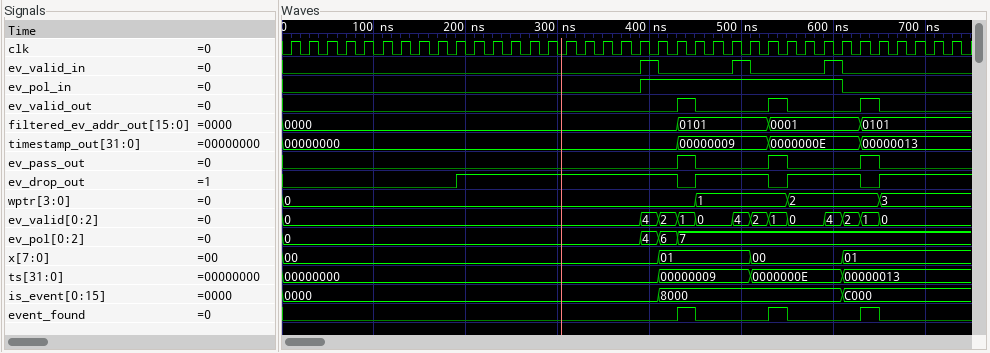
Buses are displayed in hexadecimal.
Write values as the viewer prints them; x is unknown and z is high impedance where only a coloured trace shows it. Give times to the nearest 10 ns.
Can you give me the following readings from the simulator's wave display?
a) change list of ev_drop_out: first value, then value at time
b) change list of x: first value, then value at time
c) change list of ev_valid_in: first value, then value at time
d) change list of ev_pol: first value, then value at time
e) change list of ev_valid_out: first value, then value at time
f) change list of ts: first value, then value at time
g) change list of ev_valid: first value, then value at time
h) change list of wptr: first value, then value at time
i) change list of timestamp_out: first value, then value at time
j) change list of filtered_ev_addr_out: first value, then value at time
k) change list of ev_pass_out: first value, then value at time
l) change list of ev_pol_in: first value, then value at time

0, 1 at 190 ns, 0 at 430 ns, 1 at 450 ns, 0 at 530 ns, 1 at 550 ns, 0 at 630 ns, 1 at 650 ns
00, 01 at 410 ns, 00 at 510 ns, 01 at 610 ns
0, 1 at 390 ns, 0 at 410 ns, 1 at 490 ns, 0 at 510 ns, 1 at 590 ns, 0 at 610 ns
0, 4 at 390 ns, 6 at 410 ns, 7 at 430 ns
0, 1 at 430 ns, 0 at 450 ns, 1 at 530 ns, 0 at 550 ns, 1 at 630 ns, 0 at 650 ns
00000000, 00000009 at 410 ns, 0000000E at 510 ns, 00000013 at 610 ns
0, 4 at 390 ns, 2 at 410 ns, 1 at 430 ns, 0 at 450 ns, 4 at 490 ns, 2 at 510 ns, 1 at 530 ns, 0 at 550 ns, 4 at 590 ns, 2 at 610 ns, 1 at 630 ns, 0 at 650 ns
0, 1 at 450 ns, 2 at 550 ns, 3 at 650 ns
00000000, 00000009 at 430 ns, 0000000E at 530 ns, 00000013 at 630 ns
0000, 0101 at 430 ns, 0001 at 530 ns, 0101 at 630 ns
0, 1 at 430 ns, 0 at 450 ns, 1 at 530 ns, 0 at 550 ns, 1 at 630 ns, 0 at 650 ns
0, 1 at 390 ns, 0 at 610 ns
